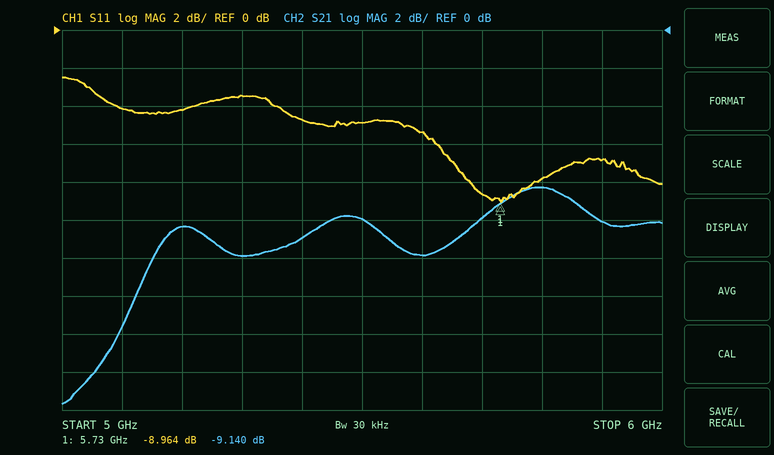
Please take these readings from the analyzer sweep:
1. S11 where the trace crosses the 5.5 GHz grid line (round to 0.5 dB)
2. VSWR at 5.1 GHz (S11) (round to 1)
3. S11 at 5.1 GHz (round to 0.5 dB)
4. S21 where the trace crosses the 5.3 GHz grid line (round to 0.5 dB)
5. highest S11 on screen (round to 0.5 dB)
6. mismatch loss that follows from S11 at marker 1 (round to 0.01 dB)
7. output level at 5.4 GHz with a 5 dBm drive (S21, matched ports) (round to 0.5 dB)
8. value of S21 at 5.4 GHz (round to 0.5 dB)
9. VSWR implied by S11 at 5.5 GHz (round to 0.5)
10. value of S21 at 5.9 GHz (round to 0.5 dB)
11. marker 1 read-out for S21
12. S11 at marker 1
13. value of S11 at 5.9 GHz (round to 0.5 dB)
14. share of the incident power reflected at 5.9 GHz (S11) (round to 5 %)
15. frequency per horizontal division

-5.0 dB
4
-4.0 dB
-12.0 dB
-2.5 dB
0.59 dB
-6.0 dBm
-11.0 dB
3.5
-10.0 dB
-9.140 dB
-8.964 dB
-7.0 dB
20 %
100 MHz
